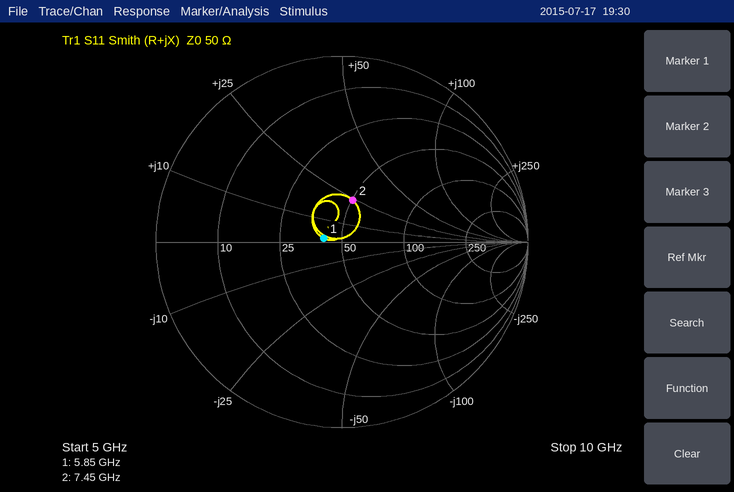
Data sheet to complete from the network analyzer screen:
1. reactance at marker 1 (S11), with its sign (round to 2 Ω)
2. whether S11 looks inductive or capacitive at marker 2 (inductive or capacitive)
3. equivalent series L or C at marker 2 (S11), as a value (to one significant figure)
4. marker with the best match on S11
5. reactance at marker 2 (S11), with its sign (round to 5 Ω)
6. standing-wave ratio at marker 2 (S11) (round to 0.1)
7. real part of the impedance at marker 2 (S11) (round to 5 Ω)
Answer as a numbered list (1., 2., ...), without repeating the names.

1. +2 Ω
2. inductive
3. 500 pH
4. marker 1
5. +25 Ω
6. 1.6
7. 50 Ω
